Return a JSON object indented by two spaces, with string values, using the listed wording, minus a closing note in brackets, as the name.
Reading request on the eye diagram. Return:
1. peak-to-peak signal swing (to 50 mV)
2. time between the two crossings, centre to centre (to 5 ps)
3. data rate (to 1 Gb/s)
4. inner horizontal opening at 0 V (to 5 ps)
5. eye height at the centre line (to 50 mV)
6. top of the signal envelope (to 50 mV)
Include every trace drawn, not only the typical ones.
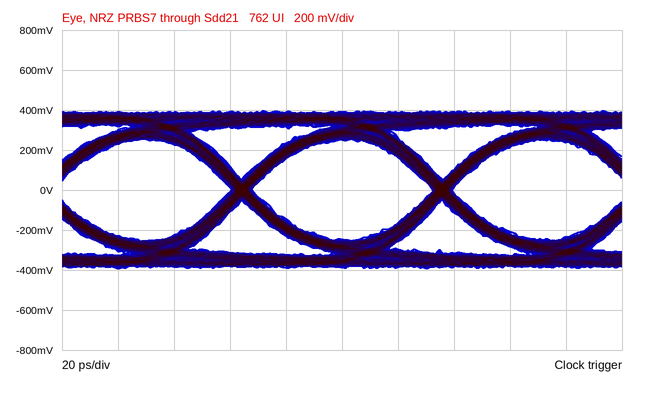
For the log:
{
  "peak-to-peak signal swing": "800 mV",
  "time between the two crossings, centre to centre": "70 ps",
  "data rate": "14 Gb/s",
  "inner horizontal opening at 0 V": "65 ps",
  "eye height at the centre line": "500 mV",
  "top of the signal envelope": "400 mV"
}
